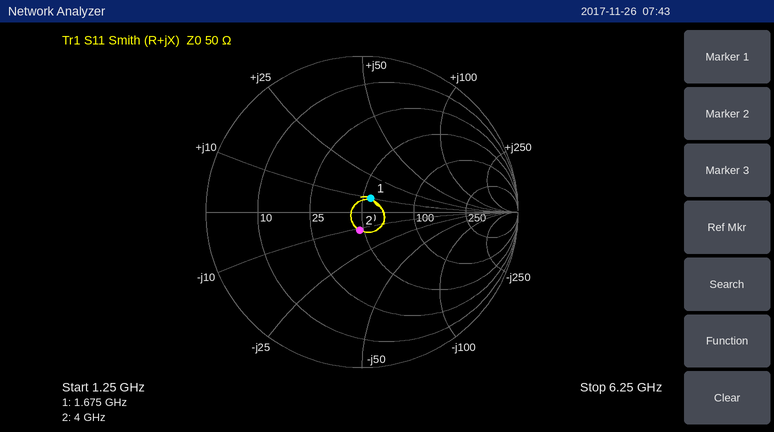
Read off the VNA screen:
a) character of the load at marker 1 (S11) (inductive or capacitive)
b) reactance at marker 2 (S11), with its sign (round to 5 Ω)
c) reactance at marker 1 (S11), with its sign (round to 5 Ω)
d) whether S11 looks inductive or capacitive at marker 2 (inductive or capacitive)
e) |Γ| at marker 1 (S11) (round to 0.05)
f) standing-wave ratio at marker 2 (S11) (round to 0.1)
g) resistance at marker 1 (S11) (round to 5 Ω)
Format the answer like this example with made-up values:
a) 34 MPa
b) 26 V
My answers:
a) inductive
b) -10 Ω
c) +10 Ω
d) capacitive
e) 0.10
f) 1.3
g) 55 Ω
